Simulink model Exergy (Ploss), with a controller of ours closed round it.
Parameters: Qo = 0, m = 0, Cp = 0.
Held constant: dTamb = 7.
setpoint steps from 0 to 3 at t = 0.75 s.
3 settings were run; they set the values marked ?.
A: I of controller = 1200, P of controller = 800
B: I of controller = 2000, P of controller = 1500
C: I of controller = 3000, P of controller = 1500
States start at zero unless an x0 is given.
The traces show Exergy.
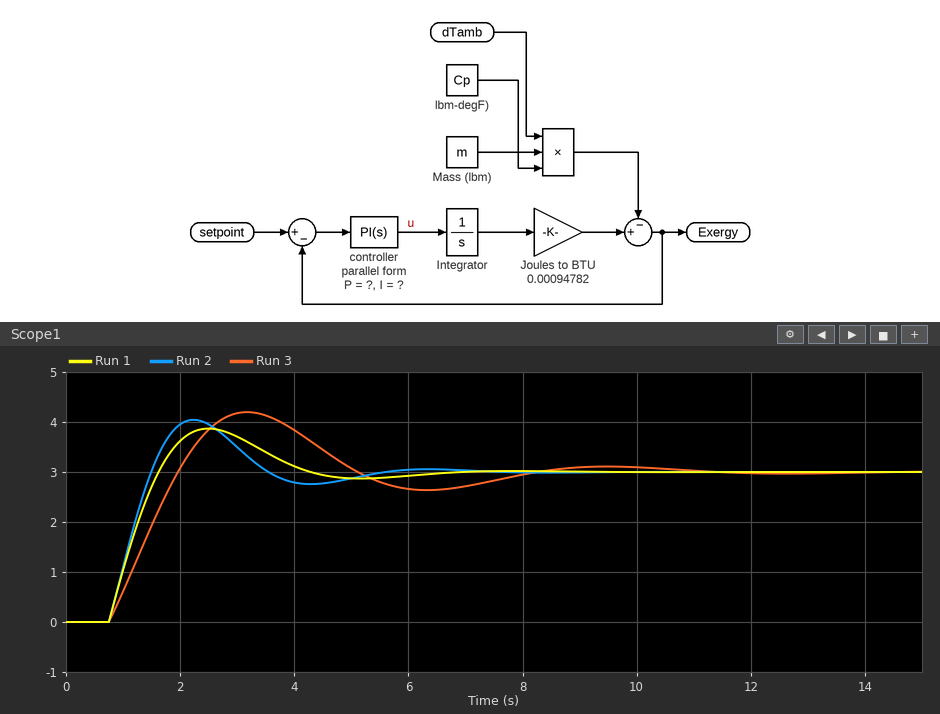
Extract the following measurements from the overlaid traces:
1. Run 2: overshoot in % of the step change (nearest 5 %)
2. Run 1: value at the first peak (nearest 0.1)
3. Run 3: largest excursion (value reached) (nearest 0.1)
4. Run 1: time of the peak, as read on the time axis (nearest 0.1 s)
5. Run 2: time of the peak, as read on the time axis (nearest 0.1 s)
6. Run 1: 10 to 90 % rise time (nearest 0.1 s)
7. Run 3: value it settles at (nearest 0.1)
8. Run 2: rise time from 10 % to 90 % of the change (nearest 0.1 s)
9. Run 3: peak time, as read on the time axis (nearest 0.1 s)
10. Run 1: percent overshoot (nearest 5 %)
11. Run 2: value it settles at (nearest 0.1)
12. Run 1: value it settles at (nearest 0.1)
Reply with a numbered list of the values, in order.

1. 35 %
2. 3.9
3. 4.2
4. 2.5 s
5. 2.2 s
6. 0.7 s
7. 3.0
8. 0.6 s
9. 3.2 s
10. 30 %
11. 3.0
12. 3.0
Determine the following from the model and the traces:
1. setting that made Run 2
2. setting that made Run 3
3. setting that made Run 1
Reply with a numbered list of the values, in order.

1. C
2. A
3. B
